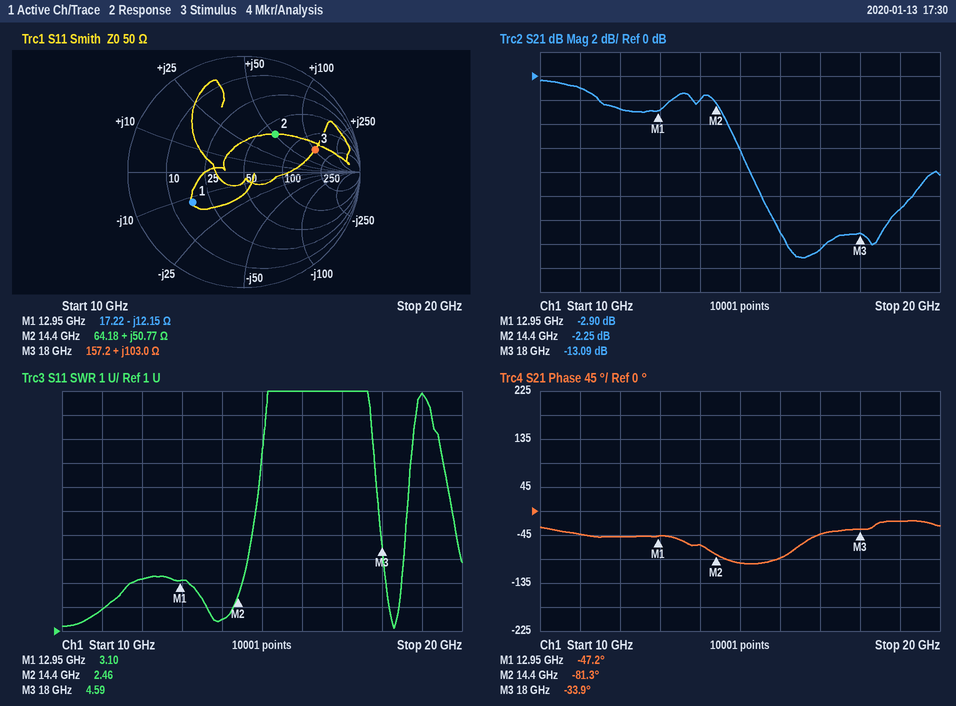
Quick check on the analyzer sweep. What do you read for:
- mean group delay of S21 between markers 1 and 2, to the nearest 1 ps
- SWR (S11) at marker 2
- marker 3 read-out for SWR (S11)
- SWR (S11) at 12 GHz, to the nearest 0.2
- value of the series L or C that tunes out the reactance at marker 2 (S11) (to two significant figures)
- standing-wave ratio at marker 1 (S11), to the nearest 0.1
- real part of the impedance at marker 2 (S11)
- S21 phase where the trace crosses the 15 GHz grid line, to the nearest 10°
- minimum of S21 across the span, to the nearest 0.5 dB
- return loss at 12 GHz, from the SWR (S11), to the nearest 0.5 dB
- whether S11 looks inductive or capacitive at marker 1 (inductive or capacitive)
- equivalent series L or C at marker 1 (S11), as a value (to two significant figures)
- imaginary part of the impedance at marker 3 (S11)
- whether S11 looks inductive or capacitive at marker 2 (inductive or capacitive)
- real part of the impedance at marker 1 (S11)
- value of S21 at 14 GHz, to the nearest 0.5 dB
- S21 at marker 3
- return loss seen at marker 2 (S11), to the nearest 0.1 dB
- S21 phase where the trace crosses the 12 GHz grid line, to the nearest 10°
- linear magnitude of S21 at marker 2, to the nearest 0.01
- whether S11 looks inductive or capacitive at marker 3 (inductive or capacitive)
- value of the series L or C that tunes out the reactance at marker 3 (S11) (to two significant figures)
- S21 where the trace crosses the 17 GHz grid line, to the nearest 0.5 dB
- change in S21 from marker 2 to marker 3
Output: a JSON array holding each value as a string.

["65 ps", "2.46", "4.59", "3.2", "220 fF", "3.1", "64.18 Ω", "-100°", "-15.0 dB", "5.5 dB", "capacitive", "1.0 pF", "+103.0 Ω", "inductive", "17.22 Ω", "-2.0 dB", "-13.09 dB", "7.5 dB", "-50°", "0.77", "inductive", "86 fF", "-14.5 dB", "-10.84 dB"]
